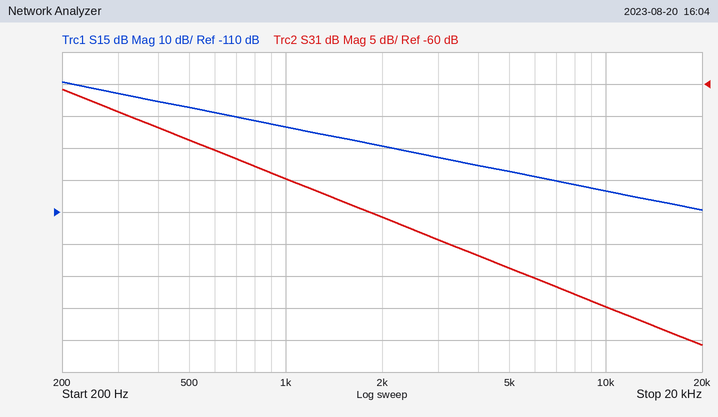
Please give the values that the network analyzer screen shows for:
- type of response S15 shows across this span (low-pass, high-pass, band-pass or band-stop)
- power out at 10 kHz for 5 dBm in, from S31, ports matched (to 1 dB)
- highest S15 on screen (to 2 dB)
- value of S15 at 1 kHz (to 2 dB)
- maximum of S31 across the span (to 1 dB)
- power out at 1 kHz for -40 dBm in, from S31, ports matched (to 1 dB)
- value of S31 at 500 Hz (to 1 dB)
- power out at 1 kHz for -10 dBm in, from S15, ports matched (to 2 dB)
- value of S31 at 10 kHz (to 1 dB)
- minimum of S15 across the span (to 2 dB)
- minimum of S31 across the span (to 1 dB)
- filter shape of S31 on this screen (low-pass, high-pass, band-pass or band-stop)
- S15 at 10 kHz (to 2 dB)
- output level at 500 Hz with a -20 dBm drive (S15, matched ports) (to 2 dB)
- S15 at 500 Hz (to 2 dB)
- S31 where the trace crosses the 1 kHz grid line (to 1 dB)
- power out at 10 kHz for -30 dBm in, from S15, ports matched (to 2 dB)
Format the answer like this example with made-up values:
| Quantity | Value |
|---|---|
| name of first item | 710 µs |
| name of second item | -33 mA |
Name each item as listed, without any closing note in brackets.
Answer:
| Quantity | Value |
|---|---|
| type of response S15 shows across this span | low-pass |
| power out at 10 kHz for 5 dBm in, from S31, ports matched | -90 dBm |
| highest S15 on screen | -70 dB |
| value of S15 at 1 kHz | -84 dB |
| maximum of S31 across the span | -61 dB |
| power out at 1 kHz for -40 dBm in, from S31, ports matched | -115 dBm |
| value of S31 at 500 Hz | -69 dB |
| power out at 1 kHz for -10 dBm in, from S15, ports matched | -94 dBm |
| value of S31 at 10 kHz | -95 dB |
| minimum of S15 across the span | -110 dB |
| minimum of S31 across the span | -101 dB |
| filter shape of S31 on this screen | low-pass |
| S15 at 10 kHz | -104 dB |
| output level at 500 Hz with a -20 dBm drive (S15, matched ports) | -98 dBm |
| S15 at 500 Hz | -78 dB |
| S31 where the trace crosses the 1 kHz grid line | -75 dB |
| power out at 10 kHz for -30 dBm in, from S15, ports matched | -134 dBm |
